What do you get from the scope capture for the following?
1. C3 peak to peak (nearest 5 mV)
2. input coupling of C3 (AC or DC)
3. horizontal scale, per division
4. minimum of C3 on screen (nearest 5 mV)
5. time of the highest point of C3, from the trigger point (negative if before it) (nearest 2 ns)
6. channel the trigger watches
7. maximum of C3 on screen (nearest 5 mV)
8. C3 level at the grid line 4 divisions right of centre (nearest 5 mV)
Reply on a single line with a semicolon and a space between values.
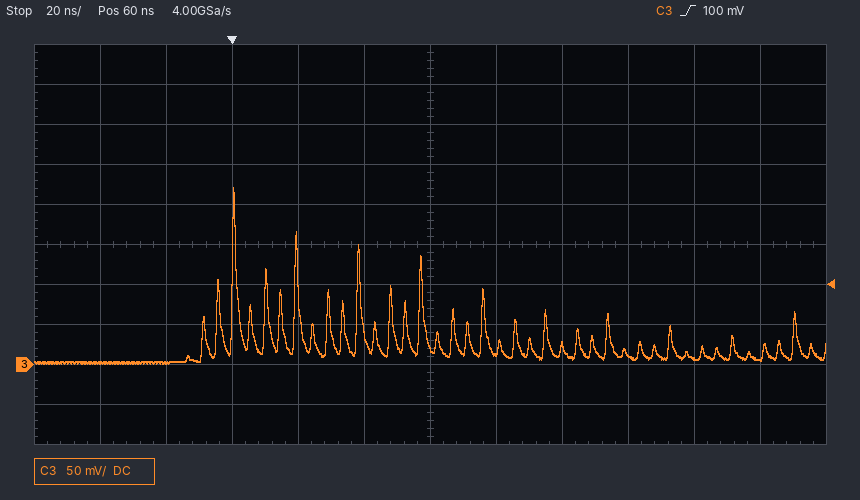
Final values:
220 mV; DC; 20 ns; 0 mV; 0 ns; C3; 220 mV; 10 mV
